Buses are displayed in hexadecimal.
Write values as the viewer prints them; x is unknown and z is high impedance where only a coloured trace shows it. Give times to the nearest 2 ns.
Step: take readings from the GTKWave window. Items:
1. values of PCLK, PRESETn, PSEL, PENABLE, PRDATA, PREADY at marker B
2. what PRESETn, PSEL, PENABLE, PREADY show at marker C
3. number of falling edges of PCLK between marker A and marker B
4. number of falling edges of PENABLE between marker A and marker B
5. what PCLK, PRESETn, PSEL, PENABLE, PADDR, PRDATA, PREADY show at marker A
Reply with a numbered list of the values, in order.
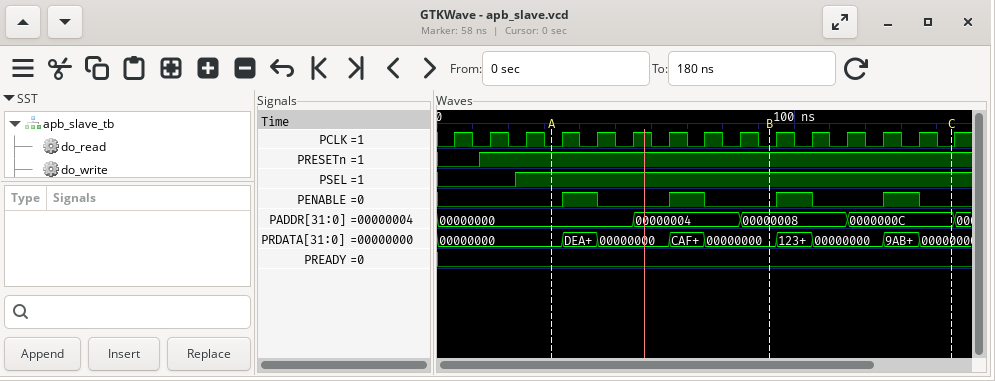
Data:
1. PCLK=0, PRESETn=1, PSEL=1, PENABLE=0, PRDATA=00000000, PREADY=0
2. PRESETn=1, PSEL=1, PENABLE=0, PREADY=0
3. 6
4. 2
5. PCLK=0, PRESETn=1, PSEL=1, PENABLE=0, PADDR=00000000, PRDATA=00000000, PREADY=0
